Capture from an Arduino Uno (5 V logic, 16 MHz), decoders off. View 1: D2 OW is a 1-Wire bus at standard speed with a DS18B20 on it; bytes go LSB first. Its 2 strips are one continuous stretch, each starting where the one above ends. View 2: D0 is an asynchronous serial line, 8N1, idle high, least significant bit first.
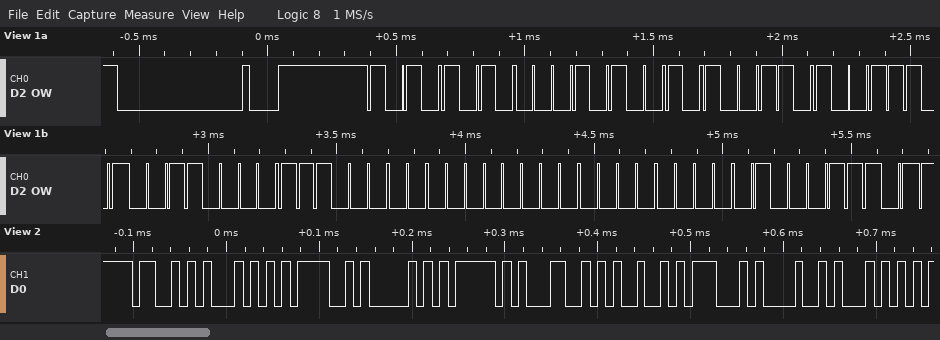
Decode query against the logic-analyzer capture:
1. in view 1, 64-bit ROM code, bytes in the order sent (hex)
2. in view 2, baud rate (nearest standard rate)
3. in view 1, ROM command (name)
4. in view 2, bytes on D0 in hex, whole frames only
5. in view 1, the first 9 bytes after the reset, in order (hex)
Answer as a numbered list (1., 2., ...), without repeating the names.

1. 28 65 B9 0C 07 00 00 E2
2. 115200 baud
3. Match ROM
4. 53 54 4F 50 5F 4C 49 47 48 54
5. 55 28 65 B9 0C 07 00 00 E2
